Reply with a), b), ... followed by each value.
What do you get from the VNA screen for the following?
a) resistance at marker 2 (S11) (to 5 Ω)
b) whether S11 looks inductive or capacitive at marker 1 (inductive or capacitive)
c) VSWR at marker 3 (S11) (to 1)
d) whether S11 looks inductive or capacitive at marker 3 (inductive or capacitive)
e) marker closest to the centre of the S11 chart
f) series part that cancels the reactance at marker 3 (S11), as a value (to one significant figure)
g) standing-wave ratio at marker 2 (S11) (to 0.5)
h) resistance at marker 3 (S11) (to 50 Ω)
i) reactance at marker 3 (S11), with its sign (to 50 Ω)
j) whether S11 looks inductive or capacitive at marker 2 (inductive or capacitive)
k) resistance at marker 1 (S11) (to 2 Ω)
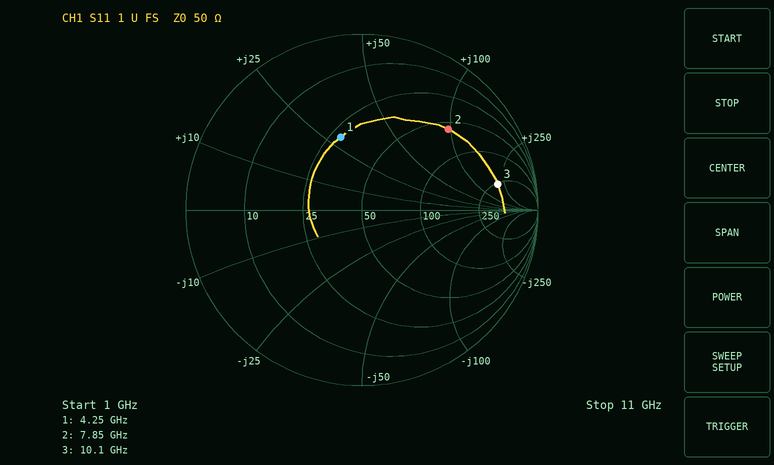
a) 60 Ω
b) inductive
c) 8
d) inductive
e) marker 1
f) 80 fF
g) 5.0
h) 250 Ω
i) +200 Ω
j) inductive
k) 28 Ω
